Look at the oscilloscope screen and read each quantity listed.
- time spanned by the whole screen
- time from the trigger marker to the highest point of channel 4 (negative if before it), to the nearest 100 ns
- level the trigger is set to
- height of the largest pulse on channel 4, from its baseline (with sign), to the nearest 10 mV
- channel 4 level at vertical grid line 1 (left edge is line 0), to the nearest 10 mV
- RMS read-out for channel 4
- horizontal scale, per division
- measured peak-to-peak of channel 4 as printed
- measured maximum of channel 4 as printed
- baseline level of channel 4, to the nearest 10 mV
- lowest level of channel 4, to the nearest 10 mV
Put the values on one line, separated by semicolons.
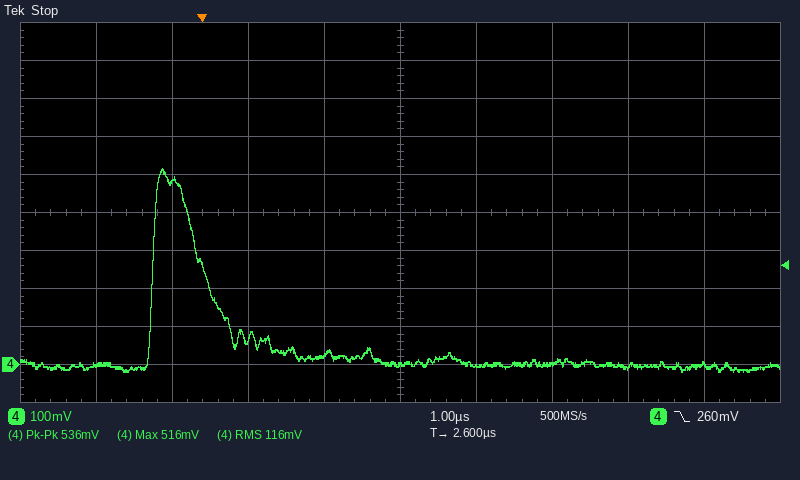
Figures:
10 µs; -500 ns; 260 mV; +520 mV; 0 mV; 116 mV; 1 µs; 536 mV; 516 mV; 0 mV; -20 mV
